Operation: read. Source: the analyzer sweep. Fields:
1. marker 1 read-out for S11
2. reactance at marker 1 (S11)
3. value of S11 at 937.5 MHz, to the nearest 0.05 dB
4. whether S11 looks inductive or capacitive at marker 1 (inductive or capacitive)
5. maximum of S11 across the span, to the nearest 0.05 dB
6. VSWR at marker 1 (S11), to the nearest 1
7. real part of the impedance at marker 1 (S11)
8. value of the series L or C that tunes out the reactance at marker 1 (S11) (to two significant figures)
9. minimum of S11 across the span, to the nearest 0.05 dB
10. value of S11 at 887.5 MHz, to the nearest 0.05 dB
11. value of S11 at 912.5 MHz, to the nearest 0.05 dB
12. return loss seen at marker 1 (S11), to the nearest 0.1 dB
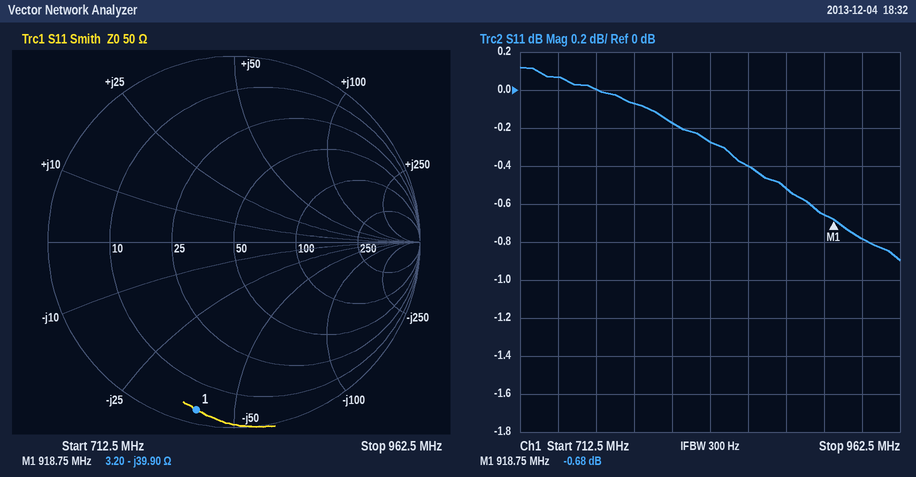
-0.68 dB
-39.90 Ω
-0.80 dB
capacitive
0.10 dB
26
3.20 Ω
6.9 nH
-0.90 dB
-0.50 dB
-0.65 dB
0.7 dB
